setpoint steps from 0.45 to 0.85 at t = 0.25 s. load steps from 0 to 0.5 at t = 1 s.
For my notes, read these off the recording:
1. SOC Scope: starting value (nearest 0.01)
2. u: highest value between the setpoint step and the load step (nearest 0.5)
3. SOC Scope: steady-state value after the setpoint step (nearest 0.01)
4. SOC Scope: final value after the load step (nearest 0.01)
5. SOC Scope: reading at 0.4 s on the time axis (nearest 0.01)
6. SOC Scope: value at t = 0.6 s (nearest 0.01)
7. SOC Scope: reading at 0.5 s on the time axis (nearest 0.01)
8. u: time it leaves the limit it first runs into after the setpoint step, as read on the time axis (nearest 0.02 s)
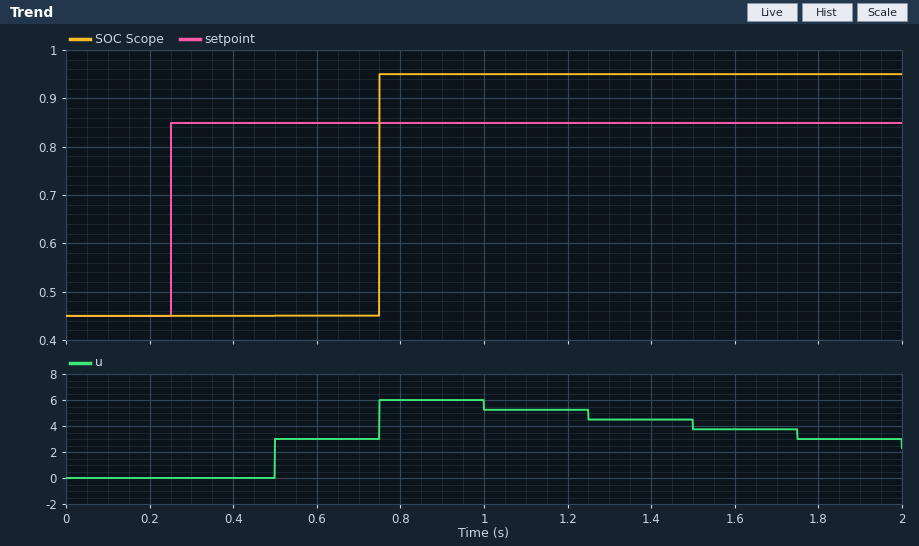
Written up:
0.45
6.0
0.95
0.95
0.45
0.45
0.45
0.50 s
